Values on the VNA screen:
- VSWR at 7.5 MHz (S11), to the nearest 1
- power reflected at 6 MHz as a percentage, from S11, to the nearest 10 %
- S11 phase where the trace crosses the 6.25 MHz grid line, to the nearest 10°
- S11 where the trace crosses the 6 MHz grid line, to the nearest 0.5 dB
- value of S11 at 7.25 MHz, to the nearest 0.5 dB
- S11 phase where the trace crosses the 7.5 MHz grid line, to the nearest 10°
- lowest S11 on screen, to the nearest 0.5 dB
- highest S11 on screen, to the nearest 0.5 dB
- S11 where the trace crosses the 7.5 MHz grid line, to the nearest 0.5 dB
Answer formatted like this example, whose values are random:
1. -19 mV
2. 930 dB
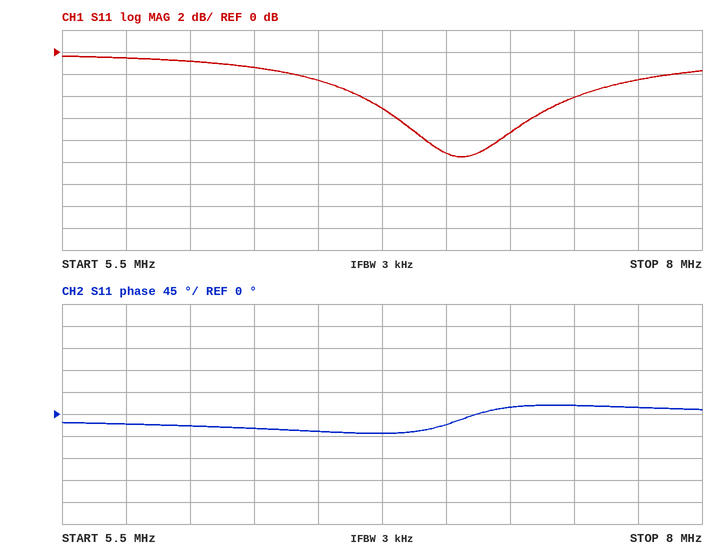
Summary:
1. 4
2. 80 %
3. -30°
4. -1.0 dB
5. -7.5 dB
6. 20°
7. -9.5 dB
8. -0.5 dB
9. -4.0 dB
